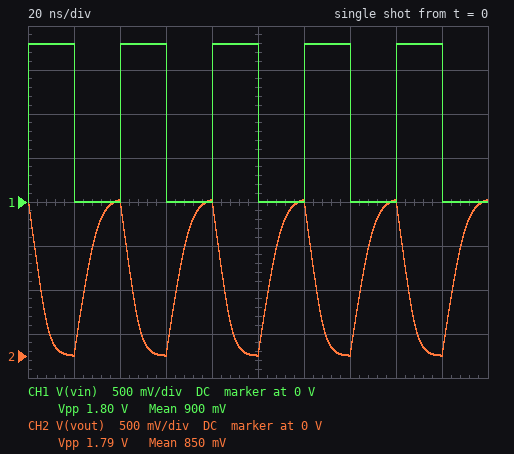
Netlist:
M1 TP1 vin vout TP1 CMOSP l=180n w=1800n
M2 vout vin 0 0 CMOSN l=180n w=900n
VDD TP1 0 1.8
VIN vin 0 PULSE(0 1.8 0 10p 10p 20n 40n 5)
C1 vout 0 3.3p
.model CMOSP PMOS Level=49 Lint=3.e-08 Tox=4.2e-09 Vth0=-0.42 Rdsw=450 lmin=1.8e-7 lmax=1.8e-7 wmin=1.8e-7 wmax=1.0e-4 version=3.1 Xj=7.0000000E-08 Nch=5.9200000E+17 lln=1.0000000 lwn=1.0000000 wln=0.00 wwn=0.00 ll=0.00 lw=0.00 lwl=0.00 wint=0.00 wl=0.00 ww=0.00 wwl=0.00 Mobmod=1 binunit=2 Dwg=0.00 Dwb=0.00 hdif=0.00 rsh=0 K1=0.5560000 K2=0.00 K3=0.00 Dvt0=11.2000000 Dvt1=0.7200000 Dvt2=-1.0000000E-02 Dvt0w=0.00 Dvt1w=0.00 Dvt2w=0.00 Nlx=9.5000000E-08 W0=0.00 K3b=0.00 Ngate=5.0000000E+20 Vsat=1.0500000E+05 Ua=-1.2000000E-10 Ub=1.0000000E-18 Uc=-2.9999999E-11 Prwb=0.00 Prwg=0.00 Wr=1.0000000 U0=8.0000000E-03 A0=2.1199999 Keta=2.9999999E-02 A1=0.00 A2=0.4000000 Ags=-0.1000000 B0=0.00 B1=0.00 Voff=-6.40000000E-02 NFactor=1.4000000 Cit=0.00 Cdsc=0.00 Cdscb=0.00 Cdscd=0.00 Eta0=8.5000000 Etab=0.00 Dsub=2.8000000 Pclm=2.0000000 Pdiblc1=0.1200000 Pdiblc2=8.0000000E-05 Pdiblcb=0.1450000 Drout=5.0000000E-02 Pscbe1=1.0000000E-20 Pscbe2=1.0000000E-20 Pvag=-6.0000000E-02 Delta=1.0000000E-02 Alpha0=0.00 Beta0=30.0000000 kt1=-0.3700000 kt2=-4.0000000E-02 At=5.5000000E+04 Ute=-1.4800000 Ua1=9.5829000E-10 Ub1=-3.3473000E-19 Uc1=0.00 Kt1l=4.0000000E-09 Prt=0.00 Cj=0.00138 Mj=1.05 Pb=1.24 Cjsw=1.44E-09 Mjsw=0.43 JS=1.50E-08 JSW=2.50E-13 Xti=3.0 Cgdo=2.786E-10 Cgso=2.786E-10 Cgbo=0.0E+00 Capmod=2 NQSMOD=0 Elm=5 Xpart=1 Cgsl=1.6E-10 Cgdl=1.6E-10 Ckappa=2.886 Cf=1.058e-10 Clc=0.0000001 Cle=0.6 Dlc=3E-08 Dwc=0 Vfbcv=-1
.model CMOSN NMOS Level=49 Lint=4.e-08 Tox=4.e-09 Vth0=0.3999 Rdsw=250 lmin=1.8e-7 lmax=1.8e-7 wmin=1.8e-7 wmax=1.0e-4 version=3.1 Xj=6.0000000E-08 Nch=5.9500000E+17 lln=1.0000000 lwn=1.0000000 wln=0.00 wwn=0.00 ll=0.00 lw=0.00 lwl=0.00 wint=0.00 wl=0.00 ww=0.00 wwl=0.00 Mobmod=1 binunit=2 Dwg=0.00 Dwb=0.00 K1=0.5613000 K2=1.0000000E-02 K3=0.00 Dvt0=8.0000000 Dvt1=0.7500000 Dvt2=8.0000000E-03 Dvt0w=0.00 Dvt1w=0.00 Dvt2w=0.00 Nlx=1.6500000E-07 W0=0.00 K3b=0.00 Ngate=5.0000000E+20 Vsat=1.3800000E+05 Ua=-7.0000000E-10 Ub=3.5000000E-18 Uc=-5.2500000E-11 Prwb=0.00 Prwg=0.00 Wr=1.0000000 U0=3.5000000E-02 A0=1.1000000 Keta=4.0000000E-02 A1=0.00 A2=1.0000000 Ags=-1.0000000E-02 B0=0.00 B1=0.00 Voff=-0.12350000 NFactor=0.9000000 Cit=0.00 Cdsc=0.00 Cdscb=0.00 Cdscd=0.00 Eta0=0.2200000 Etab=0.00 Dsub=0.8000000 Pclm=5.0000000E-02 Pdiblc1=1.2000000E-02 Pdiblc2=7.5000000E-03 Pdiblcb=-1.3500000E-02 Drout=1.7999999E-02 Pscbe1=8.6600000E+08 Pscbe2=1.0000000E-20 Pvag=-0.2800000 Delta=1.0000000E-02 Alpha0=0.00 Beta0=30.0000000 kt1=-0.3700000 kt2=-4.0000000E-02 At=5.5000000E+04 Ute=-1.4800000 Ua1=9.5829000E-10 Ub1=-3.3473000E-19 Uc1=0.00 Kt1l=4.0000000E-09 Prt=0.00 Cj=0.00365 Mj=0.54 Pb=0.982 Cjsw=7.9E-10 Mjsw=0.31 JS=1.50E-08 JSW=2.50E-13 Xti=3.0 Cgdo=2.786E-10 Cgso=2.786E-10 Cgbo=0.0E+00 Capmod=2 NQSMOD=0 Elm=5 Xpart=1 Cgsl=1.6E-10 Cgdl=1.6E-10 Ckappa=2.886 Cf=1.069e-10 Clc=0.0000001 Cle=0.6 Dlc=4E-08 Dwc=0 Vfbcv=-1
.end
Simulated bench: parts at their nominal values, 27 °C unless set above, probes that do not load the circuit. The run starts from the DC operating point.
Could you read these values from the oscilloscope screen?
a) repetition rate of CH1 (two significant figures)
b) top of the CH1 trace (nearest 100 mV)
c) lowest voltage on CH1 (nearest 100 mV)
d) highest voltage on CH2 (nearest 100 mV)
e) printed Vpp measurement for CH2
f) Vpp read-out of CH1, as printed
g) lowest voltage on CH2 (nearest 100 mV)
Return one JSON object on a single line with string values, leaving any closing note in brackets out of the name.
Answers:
{"repetition rate of CH1": "25 MHz", "top of the CH1 trace": "1.8 V", "lowest voltage on CH1": "0 V", "highest voltage on CH2": "1.8 V", "printed Vpp measurement for CH2": "1.79 V", "Vpp read-out of CH1, as printed": "1.80 V", "lowest voltage on CH2": "0 V"}
